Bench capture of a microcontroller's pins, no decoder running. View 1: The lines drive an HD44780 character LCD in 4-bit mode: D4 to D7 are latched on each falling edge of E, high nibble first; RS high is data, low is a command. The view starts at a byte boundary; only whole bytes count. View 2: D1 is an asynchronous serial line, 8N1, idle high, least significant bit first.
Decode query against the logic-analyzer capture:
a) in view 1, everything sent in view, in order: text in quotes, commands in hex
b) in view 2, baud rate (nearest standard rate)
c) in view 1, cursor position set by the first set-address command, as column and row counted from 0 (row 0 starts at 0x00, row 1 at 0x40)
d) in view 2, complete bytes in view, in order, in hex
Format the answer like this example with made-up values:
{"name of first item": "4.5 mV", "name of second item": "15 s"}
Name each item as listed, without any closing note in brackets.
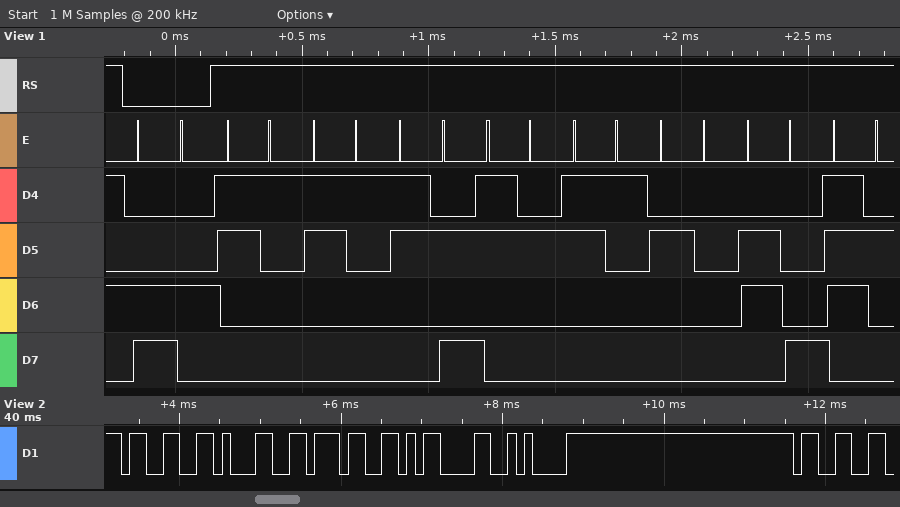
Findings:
{"in view 1, everything sent in view, in order: text in quotes, commands in hex": "0xC4 \"11:21 hr\"", "in view 2, baud rate": "9600 baud", "in view 1, cursor position set by the first set-address command, as column and row counted from 0": "column 4, row 1", "in view 2, complete bytes in view, in order, in hex": "33 31 37 0D 0A 33"}
